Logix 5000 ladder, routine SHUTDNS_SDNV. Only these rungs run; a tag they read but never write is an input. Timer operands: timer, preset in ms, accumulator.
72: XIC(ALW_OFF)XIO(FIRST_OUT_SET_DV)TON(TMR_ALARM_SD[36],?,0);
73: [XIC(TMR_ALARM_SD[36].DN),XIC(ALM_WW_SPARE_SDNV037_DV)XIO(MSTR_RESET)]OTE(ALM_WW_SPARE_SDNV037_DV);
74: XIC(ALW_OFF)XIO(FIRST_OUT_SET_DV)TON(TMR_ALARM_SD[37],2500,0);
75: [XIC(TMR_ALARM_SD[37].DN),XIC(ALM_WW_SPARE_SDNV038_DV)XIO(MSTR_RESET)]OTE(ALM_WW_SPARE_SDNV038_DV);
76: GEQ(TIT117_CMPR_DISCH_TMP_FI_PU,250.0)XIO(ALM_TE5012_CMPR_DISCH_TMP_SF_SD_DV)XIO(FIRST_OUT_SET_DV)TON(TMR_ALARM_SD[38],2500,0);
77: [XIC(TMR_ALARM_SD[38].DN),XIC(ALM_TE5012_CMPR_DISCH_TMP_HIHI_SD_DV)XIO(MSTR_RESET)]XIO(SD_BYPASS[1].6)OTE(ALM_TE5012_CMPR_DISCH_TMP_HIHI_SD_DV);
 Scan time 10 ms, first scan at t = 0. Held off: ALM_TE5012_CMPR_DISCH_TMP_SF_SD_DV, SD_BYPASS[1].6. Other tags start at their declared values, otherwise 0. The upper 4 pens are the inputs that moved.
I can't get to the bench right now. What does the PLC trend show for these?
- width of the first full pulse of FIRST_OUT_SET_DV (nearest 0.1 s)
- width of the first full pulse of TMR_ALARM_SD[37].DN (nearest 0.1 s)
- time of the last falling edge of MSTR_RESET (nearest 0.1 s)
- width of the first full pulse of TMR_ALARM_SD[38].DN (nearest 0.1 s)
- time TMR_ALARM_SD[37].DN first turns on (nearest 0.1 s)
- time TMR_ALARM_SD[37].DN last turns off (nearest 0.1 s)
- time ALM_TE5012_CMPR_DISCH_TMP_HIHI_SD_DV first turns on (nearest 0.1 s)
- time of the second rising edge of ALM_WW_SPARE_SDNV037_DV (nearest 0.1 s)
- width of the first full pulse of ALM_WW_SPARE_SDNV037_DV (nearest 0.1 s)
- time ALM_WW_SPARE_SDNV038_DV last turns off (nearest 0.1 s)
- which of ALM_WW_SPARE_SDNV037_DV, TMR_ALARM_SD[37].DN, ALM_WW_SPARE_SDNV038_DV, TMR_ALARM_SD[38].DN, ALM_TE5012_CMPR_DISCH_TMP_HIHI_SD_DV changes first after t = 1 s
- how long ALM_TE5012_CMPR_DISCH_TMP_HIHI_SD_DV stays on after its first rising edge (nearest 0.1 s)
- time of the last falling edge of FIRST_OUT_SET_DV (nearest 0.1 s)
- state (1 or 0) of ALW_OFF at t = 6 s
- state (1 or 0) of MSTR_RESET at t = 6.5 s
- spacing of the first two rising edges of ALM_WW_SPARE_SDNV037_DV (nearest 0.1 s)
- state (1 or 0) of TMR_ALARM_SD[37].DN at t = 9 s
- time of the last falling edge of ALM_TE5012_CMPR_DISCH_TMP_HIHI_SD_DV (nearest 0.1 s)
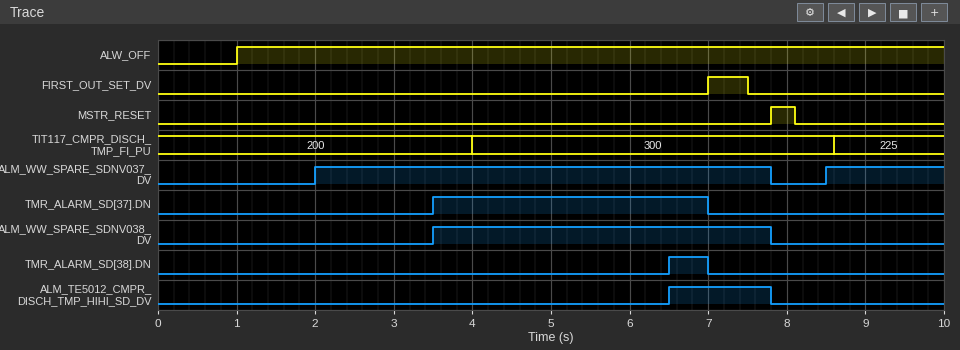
0.5 s
3.5 s
8.1 s
0.5 s
3.5 s
7.0 s
6.5 s
8.5 s
5.8 s
7.8 s
ALM_WW_SPARE_SDNV037_DV
1.3 s
7.5 s
1
0
6.5 s
0
7.8 s
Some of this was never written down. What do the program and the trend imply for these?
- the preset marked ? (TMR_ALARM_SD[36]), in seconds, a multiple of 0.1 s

1.0 s
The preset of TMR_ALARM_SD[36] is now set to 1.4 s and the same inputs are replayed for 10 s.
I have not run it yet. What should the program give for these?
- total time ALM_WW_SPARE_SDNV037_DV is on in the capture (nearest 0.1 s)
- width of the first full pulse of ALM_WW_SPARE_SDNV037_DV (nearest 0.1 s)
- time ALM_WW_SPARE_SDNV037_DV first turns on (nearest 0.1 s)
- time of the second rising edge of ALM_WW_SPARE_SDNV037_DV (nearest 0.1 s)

6.5 s
5.4 s
2.4 s
8.9 s
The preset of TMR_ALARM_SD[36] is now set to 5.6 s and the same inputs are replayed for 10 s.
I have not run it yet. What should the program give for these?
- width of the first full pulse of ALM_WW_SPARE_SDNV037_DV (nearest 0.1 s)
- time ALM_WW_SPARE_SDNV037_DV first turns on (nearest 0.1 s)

1.2 s
6.6 s
